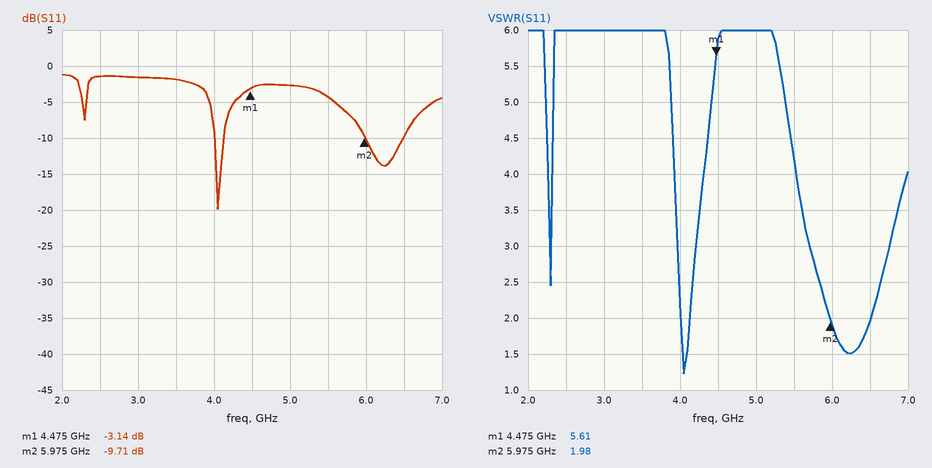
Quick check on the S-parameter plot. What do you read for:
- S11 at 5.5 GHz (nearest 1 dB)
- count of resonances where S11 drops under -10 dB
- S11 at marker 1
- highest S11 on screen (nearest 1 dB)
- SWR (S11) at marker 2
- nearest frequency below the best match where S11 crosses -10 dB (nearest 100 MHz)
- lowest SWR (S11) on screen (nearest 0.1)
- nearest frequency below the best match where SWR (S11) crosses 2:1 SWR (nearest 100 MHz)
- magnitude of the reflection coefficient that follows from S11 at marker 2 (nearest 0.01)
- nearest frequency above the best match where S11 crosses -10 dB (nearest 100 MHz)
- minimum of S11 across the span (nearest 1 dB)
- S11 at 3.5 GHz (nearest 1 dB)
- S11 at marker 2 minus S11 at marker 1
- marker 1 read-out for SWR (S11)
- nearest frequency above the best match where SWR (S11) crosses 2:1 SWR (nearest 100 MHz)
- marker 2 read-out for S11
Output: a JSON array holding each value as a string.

["-4 dB", "2", "-3.14 dB", "-1 dB", "1.98", "4.0 GHz", "1.2", "4.0 GHz", "0.33", "4.1 GHz", "-20 dB", "-2 dB", "-6.57 dB", "5.61", "4.1 GHz", "-9.71 dB"]
